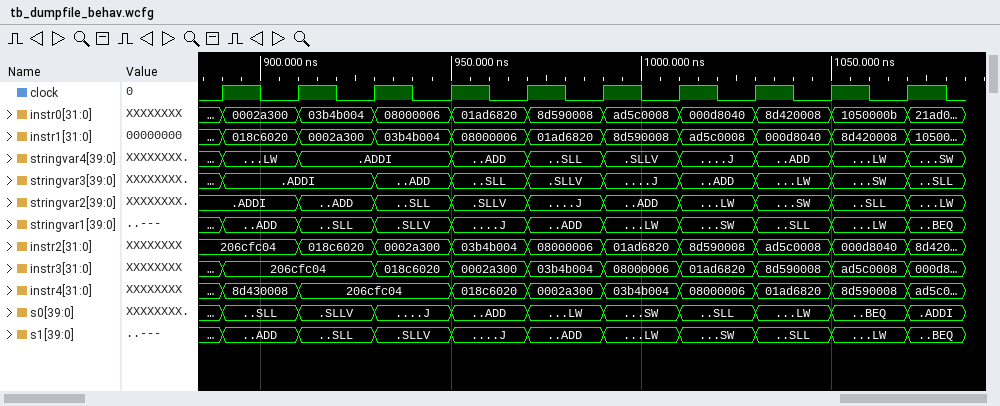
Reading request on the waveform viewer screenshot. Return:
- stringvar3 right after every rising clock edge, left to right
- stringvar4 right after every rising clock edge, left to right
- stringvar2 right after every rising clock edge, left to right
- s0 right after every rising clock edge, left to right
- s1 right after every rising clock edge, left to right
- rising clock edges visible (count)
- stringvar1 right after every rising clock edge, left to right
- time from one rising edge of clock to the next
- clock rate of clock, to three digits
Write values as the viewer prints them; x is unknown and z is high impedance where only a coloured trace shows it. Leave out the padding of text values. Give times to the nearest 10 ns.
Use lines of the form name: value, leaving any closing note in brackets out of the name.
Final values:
stringvar3 right after every rising clock edge, left to right: ADDI, ADDI, ADD, SLL, SLLV, J, ADD, LW, SW, SLL
stringvar4 right after every rising clock edge, left to right: LW, ADDI, ADDI, ADD, SLL, SLLV, J, ADD, LW, SW
stringvar2 right after every rising clock edge, left to right: ADDI, ADD, SLL, SLLV, J, ADD, LW, SW, SLL, LW
s0 right after every rising clock edge, left to right: SLL, SLLV, J, ADD, LW, SW, SLL, LW, BEQ, ADDI
s1 right after every rising clock edge, left to right: ADD, SLL, SLLV, J, ADD, LW, SW, SLL, LW, BEQ
rising clock edges visible: 10
stringvar1 right after every rising clock edge, left to right: ADD, SLL, SLLV, J, ADD, LW, SW, SLL, LW, BEQ
time from one rising edge of clock to the next: 20 ns
clock rate of clock, to three digits: 50.0 MHz
